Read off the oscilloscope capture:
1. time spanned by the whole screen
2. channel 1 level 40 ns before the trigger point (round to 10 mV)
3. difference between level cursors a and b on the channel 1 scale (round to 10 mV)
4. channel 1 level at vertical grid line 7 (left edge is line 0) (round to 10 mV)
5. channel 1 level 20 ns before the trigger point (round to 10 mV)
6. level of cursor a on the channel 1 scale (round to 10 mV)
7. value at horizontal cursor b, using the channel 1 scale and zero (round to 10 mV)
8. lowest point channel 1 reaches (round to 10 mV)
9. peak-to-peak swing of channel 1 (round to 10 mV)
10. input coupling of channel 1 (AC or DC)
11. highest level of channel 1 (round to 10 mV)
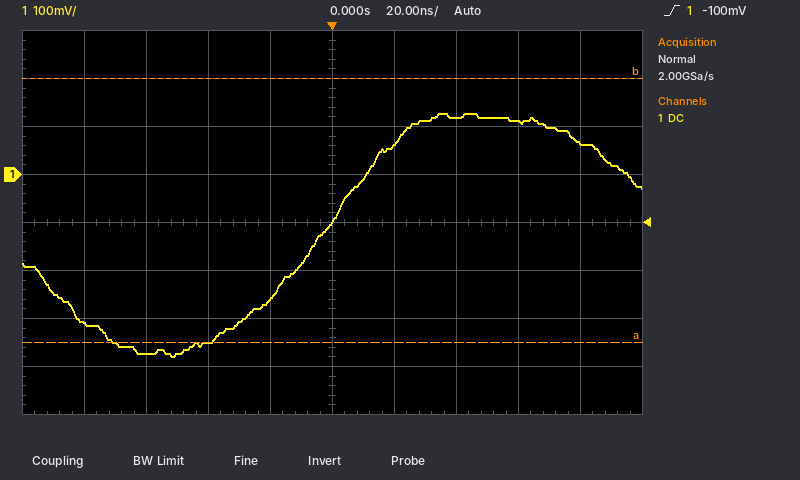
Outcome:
200 ns
-350 mV
550 mV
120 mV
-260 mV
-350 mV
200 mV
-380 mV
510 mV
DC
130 mV
